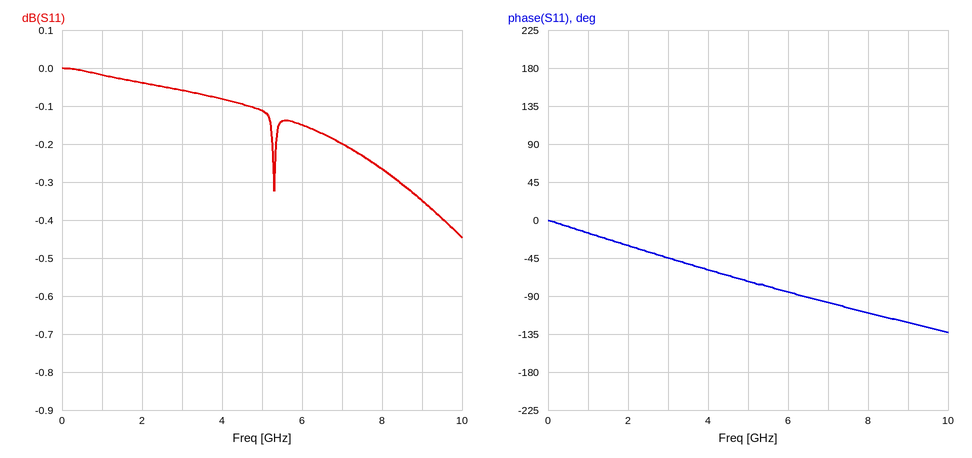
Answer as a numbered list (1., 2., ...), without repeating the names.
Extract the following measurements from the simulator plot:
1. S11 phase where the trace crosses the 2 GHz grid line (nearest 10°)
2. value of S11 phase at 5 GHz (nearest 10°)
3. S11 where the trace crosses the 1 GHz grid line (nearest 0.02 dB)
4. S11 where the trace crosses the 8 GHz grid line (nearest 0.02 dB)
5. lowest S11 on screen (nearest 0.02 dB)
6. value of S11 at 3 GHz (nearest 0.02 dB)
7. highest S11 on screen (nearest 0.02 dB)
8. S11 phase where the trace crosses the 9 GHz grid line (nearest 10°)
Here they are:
1. -30°
2. -70°
3. -0.02 dB
4. -0.26 dB
5. -0.44 dB
6. -0.06 dB
7. 0.00 dB
8. -120°
